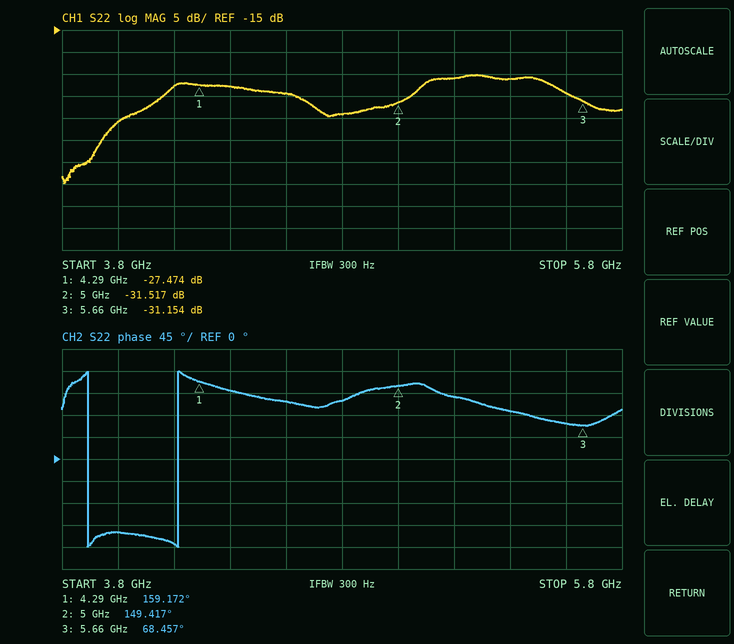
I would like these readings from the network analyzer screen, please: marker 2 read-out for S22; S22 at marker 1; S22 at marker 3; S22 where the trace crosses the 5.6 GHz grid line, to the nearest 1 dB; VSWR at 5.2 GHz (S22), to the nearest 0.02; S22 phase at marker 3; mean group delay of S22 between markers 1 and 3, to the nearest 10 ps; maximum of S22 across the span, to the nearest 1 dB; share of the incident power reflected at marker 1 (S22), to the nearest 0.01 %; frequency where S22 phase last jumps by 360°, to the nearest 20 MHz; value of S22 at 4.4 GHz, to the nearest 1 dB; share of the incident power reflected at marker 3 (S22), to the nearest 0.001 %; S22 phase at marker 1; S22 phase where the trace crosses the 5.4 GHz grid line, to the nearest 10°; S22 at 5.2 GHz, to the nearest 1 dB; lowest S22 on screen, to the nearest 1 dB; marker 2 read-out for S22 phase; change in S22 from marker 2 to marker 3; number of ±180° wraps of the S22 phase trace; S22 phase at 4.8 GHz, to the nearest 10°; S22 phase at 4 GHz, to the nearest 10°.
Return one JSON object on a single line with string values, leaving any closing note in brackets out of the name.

{"marker 2 read-out for S22": "-31.517 dB", "S22 at marker 1": "-27.474 dB", "S22 at marker 3": "-31.154 dB", "S22 where the trace crosses the 5.6 GHz grid line, to the nearest 1 dB": "-29 dB", "VSWR at 5.2 GHz (S22), to the nearest 0.02": "1.10", "S22 phase at marker 3": "68.457°", "mean group delay of S22 between markers 1 and 3, to the nearest 10 ps": "180 ps", "maximum of S22 across the span, to the nearest 1 dB": "-25 dB", "share of the incident power reflected at marker 1 (S22), to the nearest 0.01 %": "0.18 %", "frequency where S22 phase last jumps by 360°, to the nearest 20 MHz": "4.22 GHz", "value of S22 at 4.4 GHz, to the nearest 1 dB": "-28 dB", "share of the incident power reflected at marker 3 (S22), to the nearest 0.001 %": "0.077 %", "S22 phase at marker 1": "159.172°", "S22 phase where the trace crosses the 5.4 GHz grid line, to the nearest 10°": "100°", "S22 at 5.2 GHz, to the nearest 1 dB": "-26 dB", "lowest S22 on screen, to the nearest 1 dB": "-50 dB", "marker 2 read-out for S22 phase": "149.417°", "change in S22 from marker 2 to marker 3": "0.363 dB", "number of ±180° wraps of the S22 phase trace": "2", "S22 phase at 4.8 GHz, to the nearest 10°": "120°", "S22 phase at 4 GHz, to the nearest 10°": "-150°"}
